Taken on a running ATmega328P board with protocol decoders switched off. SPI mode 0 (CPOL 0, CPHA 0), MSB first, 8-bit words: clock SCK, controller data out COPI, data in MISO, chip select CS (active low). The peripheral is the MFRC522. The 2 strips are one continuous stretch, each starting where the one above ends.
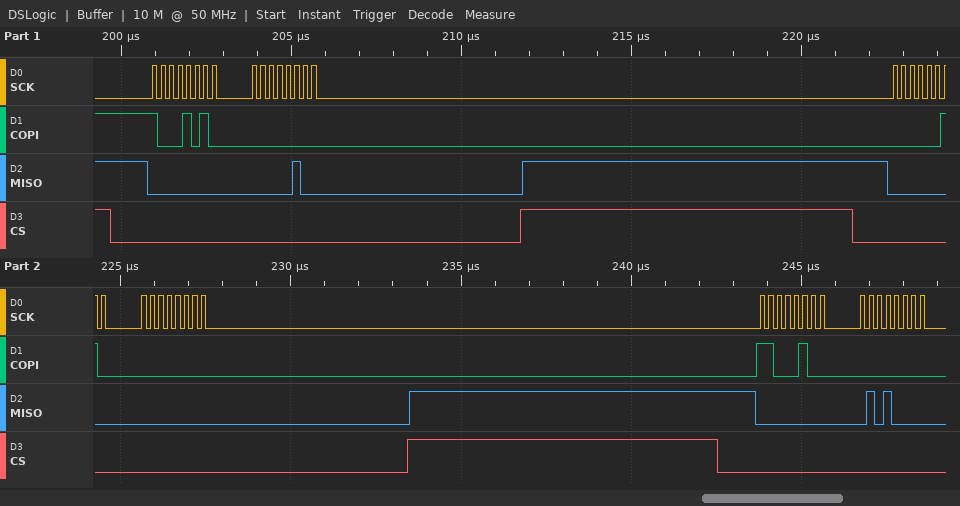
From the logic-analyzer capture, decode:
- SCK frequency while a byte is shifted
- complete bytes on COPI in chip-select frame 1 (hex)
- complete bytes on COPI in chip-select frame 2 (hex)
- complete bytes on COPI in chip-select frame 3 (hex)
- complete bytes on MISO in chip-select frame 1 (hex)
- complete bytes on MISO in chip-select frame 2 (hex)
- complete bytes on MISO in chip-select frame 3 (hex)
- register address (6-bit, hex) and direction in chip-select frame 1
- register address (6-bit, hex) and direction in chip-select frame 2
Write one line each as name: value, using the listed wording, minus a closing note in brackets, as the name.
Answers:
SCK frequency while a byte is shifted: 4 MHz
complete bytes on COPI in chip-select frame 1: 8A 00
complete bytes on COPI in chip-select frame 2: 02 00
complete bytes on COPI in chip-select frame 3: C4 00
complete bytes on MISO in chip-select frame 1: 00 04
complete bytes on MISO in chip-select frame 2: 00 00
complete bytes on MISO in chip-select frame 3: 00 50
register address (6-bit, hex) and direction in chip-select frame 1: 0x05 read
register address (6-bit, hex) and direction in chip-select frame 2: 0x01 write
